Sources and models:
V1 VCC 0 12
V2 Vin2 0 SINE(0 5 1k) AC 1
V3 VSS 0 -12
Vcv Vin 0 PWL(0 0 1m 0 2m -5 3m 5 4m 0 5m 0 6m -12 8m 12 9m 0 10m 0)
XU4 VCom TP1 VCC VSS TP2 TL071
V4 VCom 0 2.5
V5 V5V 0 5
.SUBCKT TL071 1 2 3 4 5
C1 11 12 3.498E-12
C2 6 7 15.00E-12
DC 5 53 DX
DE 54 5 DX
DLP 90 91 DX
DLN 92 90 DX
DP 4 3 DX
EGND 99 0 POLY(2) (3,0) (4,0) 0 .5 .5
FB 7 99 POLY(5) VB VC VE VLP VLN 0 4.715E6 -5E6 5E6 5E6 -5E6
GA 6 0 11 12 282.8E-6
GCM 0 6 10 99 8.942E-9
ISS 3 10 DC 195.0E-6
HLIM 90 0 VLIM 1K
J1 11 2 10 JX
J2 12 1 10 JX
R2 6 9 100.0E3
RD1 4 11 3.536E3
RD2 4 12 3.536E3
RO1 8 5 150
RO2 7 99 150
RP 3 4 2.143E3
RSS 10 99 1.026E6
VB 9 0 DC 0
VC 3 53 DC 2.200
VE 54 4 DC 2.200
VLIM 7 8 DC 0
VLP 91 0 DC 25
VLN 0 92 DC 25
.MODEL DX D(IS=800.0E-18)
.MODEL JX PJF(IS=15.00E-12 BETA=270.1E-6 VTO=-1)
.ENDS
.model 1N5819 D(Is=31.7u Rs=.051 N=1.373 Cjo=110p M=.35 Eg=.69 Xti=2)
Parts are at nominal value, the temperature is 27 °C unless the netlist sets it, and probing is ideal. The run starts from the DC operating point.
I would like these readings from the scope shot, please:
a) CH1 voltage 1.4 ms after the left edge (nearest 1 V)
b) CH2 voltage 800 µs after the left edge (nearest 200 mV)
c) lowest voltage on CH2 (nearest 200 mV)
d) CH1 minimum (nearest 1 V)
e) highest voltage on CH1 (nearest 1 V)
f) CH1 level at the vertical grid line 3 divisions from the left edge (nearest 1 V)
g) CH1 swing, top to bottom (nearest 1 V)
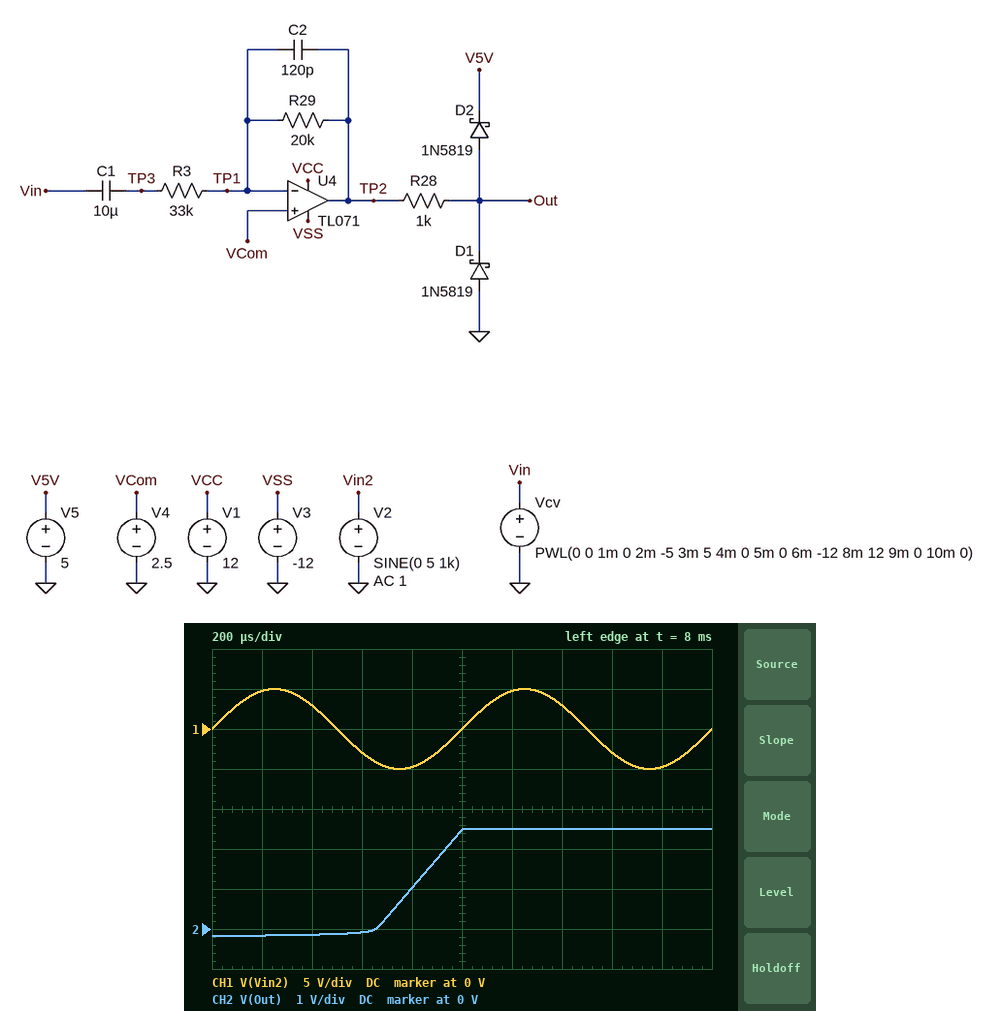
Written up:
3 V
1.0 V
-200 mV
-5 V
5 V
-3 V
10 V
